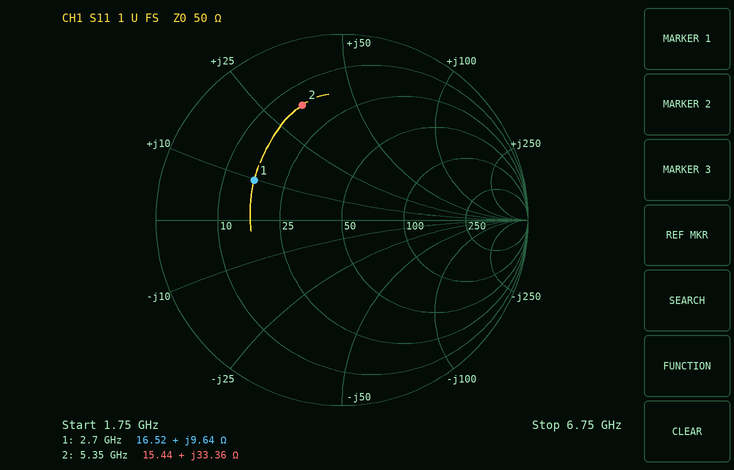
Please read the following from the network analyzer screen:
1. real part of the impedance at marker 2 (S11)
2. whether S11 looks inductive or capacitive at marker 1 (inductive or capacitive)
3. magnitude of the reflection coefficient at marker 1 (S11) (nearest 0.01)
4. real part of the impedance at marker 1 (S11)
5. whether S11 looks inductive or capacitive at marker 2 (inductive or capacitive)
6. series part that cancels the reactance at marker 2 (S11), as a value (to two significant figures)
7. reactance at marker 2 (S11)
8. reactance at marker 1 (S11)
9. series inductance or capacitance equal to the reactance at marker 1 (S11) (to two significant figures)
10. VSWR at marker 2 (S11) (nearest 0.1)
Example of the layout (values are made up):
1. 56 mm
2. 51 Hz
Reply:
1. 15.44 Ω
2. inductive
3. 0.52
4. 16.52 Ω
5. inductive
6. 890 fF
7. +33.36 Ω
8. +9.64 Ω
9. 570 pH
10. 4.8
